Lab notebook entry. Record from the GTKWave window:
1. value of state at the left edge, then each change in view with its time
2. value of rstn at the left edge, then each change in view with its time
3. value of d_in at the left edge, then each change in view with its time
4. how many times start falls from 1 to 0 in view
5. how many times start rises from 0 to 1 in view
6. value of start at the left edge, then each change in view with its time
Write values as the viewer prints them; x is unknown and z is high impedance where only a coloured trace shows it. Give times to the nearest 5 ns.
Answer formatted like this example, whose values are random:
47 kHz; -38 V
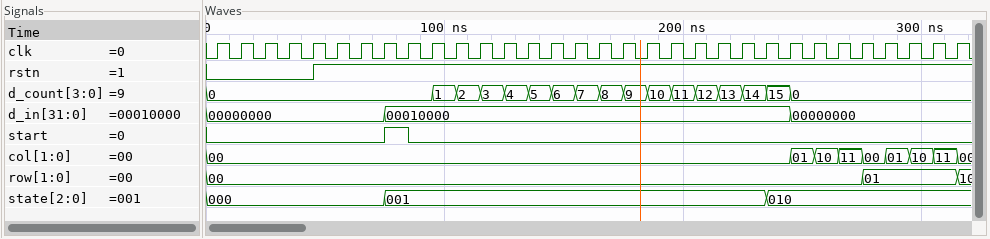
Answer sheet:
000, 001 at 75 ns, 010 at 235 ns; 0, 1 at 45 ns; 00000000, 00010000 at 75 ns, 00000000 at 245 ns; 1; 1; 0, 1 at 75 ns, 0 at 85 ns
